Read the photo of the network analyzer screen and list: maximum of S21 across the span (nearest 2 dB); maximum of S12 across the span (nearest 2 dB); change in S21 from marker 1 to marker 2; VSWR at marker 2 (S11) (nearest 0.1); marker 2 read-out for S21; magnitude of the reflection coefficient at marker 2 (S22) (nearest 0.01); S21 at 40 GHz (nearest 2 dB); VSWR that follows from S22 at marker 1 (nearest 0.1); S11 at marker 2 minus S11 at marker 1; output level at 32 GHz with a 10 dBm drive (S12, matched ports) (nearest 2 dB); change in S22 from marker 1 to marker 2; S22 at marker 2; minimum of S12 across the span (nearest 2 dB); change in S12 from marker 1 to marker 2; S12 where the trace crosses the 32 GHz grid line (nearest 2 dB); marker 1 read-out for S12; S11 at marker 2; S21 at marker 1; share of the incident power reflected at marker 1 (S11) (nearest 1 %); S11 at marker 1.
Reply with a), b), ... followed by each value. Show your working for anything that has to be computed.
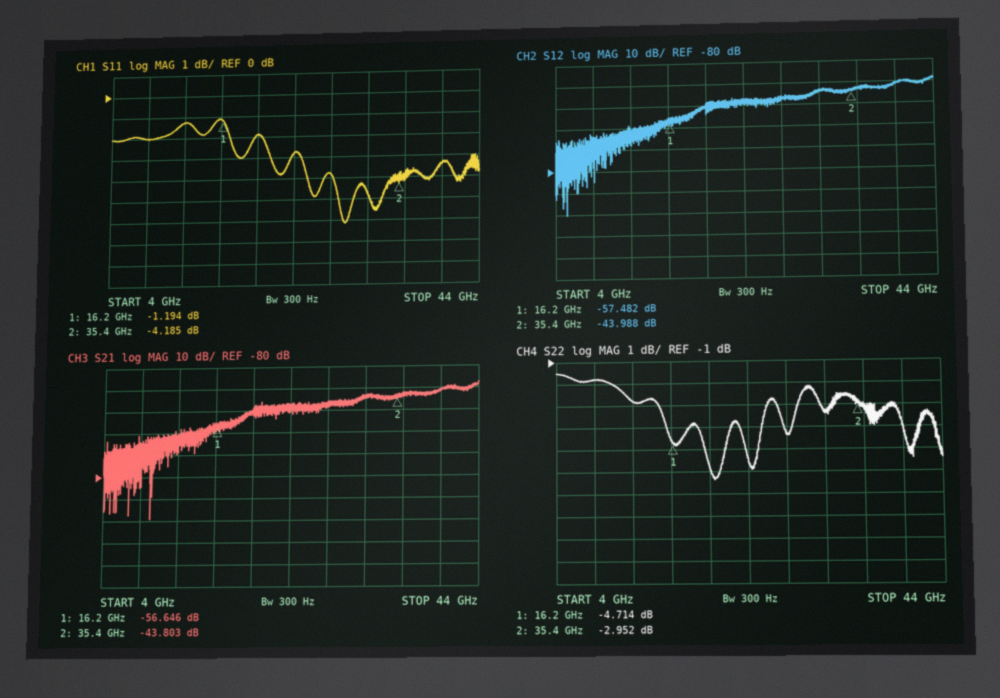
a) -38 dB
b) -38 dB
c) -43.803 − (-56.646) = 12.843 dB
d) (1 + 0.6177)/(1 − 0.6177) ≈ 4.2
e) -43.803 dB
f) 10^(-2.952/20) ≈ 0.71
g) -42 dB
h) (1 + 0.5812)/(1 − 0.5812) ≈ 3.8
i) -4.185 − (-1.194) = -2.991 dB
j) 10 dBm + (-44 dB) = -34 dBm
k) -2.952 − (-4.714) = 1.762 dB
l) -2.952 dB
m) -100 dB
n) -43.988 − (-57.482) = 13.494 dB
o) -44 dB
p) -57.482 dB
q) -4.185 dB
r) -56.646 dB
s) 10^(-1.194/10) ≈ 76 %
t) -1.194 dB
